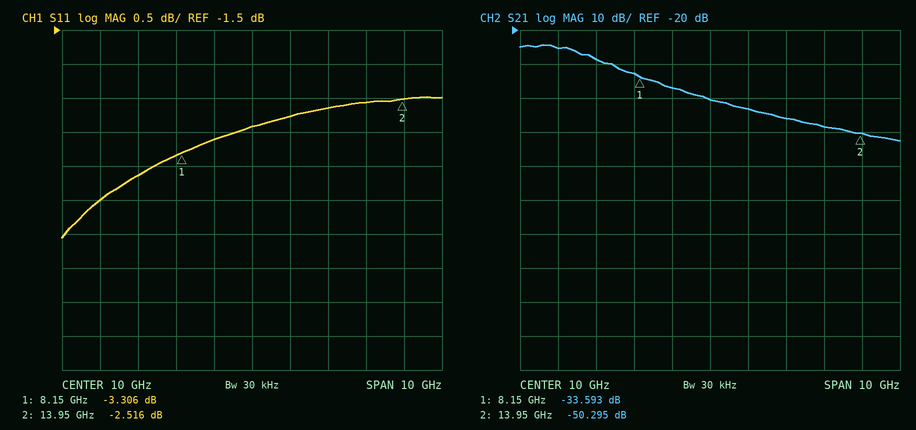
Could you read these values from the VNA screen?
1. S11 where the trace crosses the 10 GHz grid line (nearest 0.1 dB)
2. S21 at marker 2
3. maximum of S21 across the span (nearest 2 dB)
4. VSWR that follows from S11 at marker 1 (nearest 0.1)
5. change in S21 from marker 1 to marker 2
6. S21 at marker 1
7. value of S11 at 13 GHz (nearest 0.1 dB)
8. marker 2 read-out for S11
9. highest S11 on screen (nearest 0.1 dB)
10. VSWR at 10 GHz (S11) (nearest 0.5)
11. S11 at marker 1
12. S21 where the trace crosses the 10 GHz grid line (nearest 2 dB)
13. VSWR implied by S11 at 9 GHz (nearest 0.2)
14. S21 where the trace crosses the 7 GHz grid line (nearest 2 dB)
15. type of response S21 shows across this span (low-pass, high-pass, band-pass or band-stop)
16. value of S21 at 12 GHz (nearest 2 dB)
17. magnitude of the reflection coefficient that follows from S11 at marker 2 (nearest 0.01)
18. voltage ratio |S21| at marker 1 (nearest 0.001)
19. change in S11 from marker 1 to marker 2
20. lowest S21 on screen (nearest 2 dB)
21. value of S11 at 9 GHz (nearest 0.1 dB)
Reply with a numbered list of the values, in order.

1. -2.9 dB
2. -50.295 dB
3. -24 dB
4. 5.3
5. -16.702 dB
6. -33.593 dB
7. -2.6 dB
8. -2.516 dB
9. -2.5 dB
10. 6.0
11. -3.306 dB
12. -40 dB
13. 5.6
14. -28 dB
15. low-pass
16. -46 dB
17. 0.75
18. 0.021
19. 0.790 dB
20. -52 dB
21. -3.1 dB
